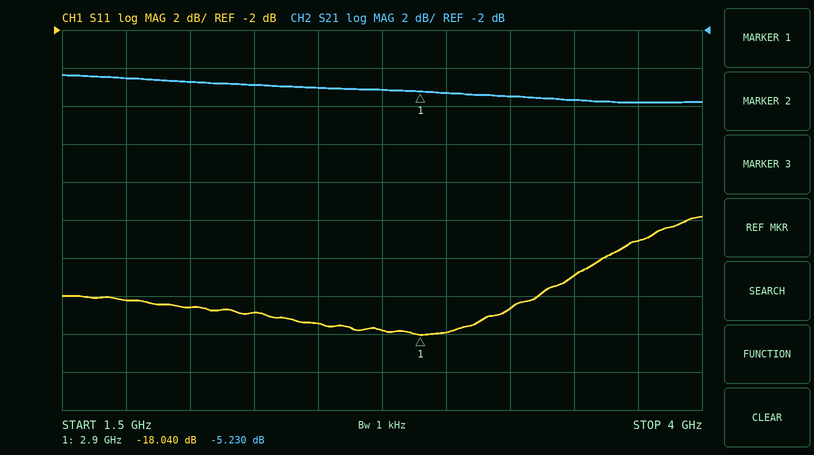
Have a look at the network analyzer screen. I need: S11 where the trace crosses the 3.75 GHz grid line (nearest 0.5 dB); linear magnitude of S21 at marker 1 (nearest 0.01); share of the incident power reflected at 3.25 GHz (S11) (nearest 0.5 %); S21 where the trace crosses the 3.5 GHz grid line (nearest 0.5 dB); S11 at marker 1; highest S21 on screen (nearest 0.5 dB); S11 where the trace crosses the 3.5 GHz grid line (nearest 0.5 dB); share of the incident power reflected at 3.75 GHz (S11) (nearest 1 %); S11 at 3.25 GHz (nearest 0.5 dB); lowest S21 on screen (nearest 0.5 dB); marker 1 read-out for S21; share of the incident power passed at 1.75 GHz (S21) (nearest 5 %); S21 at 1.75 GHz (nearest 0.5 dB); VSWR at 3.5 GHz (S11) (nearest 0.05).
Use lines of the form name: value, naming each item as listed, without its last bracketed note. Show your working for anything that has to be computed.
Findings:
S11 where the trace crosses the 3.75 GHz grid line: -13.0 dB
linear magnitude of S21 at marker 1: 10^(-5.23/20) ≈ 0.55
share of the incident power reflected at 3.25 GHz (S11): 10^(-16.5/10) ≈ 2.24 %, so 2.0 % to the nearest 0.5 %
S21 where the trace crosses the 3.5 GHz grid line: -5.5 dB
S11 at marker 1: -18.040 dB
highest S21 on screen: -4.5 dB
S11 where the trace crosses the 3.5 GHz grid line: -15.0 dB
share of the incident power reflected at 3.75 GHz (S11): 10^(-13/10) ≈ 5 %
S11 at 3.25 GHz: -16.5 dB
lowest S21 on screen: -6.0 dB
marker 1 read-out for S21: -5.230 dB
share of the incident power passed at 1.75 GHz (S21): 10^(-4.5/10) ≈ 35 %
S21 at 1.75 GHz: -4.5 dB
VSWR at 3.5 GHz (S11): |Γ| = 10^(-15/20) = 0.1778; VSWR = (1 + 0.1778)/(1 − 0.1778) ≈ 1.43, so 1.45 to the nearest 0.05
